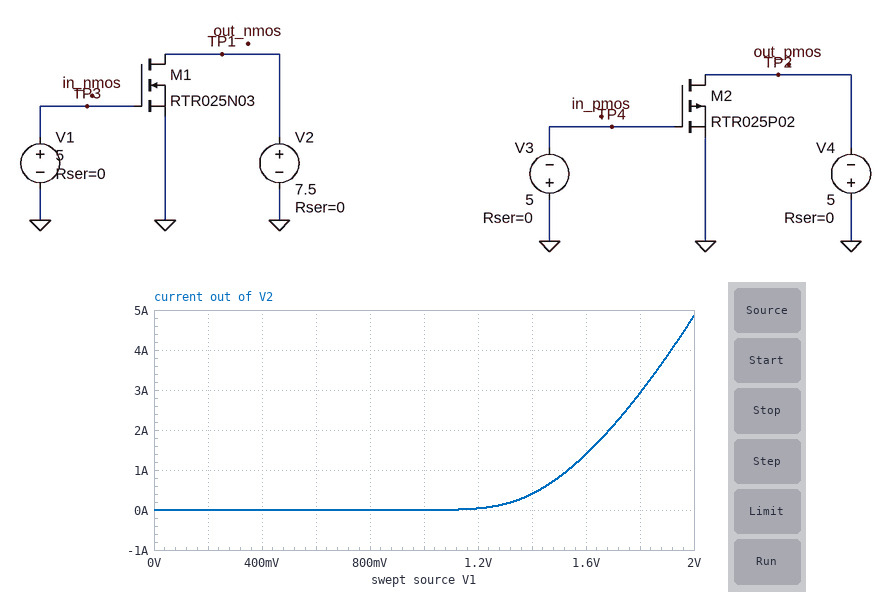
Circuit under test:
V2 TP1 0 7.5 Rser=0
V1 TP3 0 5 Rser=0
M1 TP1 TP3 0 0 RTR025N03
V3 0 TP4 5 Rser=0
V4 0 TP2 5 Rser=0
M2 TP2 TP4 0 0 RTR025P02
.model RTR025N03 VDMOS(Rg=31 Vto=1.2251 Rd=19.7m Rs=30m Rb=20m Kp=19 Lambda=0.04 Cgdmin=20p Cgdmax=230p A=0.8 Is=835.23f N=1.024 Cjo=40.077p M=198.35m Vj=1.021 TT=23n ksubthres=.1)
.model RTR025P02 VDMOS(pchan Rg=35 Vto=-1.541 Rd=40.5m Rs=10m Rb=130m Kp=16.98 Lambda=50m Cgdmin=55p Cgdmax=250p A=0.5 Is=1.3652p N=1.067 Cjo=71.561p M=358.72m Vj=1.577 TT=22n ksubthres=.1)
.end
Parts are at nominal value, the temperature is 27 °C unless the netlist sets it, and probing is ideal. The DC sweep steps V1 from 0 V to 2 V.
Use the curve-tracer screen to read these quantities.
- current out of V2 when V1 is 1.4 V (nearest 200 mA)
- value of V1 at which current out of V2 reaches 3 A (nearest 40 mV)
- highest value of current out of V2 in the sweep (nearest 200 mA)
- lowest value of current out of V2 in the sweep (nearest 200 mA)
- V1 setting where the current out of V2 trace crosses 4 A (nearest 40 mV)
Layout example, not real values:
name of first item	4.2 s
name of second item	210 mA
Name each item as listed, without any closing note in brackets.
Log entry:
current out of V2 when V1 is 1.4 V	400 mA
value of V1 at which current out of V2 reaches 3 A	1.80 V
highest value of current out of V2 in the sweep	4.8 A
lowest value of current out of V2 in the sweep	0 A
V1 setting where the current out of V2 trace crosses 4 A	1.92 V
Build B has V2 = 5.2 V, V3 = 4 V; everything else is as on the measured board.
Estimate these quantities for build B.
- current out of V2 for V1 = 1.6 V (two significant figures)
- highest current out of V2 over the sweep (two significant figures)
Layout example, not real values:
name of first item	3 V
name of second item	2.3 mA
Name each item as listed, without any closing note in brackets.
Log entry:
current out of V2 for V1 = 1.6 V	1.3 A
highest current out of V2 over the sweep	4.6 A
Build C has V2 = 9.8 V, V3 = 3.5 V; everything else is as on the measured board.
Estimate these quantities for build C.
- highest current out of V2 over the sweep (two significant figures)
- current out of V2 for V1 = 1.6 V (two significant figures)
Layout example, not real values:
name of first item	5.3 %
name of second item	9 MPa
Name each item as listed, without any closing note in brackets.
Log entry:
highest current out of V2 over the sweep	5.1 A
current out of V2 for V1 = 1.6 V	1.5 A
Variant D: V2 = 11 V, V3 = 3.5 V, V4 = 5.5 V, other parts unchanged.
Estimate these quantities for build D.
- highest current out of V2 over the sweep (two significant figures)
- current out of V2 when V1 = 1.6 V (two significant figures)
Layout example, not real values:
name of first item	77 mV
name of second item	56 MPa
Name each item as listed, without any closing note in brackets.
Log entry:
highest current out of V2 over the sweep	5.2 A
current out of V2 when V1 = 1.6 V	1.5 A
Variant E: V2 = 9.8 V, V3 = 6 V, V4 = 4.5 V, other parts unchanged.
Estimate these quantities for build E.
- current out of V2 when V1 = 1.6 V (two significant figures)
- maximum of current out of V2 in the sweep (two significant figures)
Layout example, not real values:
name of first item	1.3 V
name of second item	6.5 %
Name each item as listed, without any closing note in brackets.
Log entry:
current out of V2 when V1 = 1.6 V	1.5 A
maximum of current out of V2 in the sweep	5.1 A
